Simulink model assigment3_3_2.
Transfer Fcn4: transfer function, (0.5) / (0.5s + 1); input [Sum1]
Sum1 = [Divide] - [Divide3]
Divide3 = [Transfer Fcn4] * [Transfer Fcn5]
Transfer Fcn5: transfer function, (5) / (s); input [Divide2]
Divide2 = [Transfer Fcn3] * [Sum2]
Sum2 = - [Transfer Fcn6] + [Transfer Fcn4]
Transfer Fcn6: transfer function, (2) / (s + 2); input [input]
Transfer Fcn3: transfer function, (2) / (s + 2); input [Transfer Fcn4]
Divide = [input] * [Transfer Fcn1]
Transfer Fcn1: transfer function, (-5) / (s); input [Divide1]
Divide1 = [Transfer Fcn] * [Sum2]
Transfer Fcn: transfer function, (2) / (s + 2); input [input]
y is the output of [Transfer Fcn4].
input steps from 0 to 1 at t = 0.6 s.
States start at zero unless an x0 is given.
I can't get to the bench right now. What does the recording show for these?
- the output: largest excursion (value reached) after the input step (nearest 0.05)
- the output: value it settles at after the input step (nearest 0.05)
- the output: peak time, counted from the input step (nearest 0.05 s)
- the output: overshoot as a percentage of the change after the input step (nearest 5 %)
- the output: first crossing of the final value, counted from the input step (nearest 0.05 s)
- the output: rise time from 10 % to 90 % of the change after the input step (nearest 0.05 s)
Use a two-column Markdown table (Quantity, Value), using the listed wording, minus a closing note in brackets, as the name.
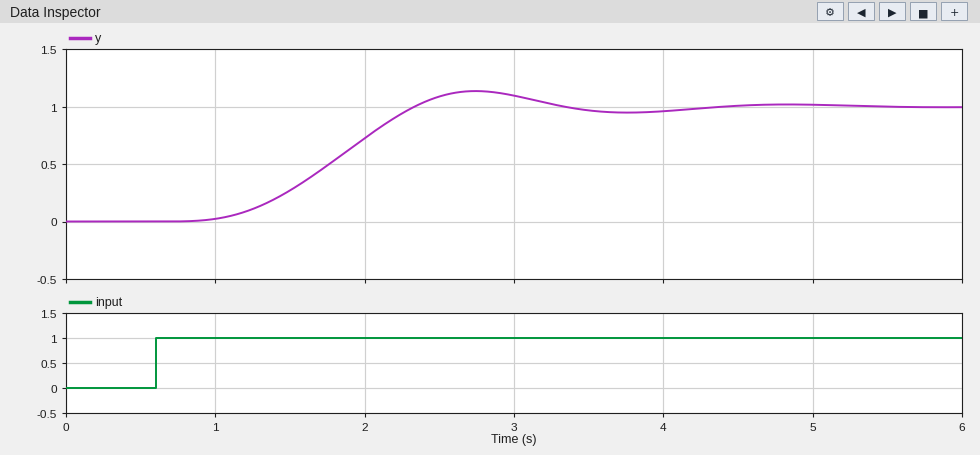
| Quantity | Value |
|---|---|
| the output: largest excursion (value reached) after the input step | 1.15 |
| the output: value it settles at after the input step | 1.00 |
| the output: peak time, counted from the input step | 2.15 s |
| the output: overshoot as a percentage of the change after the input step | 15 % |
| the output: first crossing of the final value, counted from the input step | 1.75 s |
| the output: rise time from 10 % to 90 % of the change after the input step | 0.95 s |
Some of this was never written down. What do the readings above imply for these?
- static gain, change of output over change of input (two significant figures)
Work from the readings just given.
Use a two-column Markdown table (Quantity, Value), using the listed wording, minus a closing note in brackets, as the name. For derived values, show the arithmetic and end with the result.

| Quantity | Value |
|---|---|
| static gain, change of output over change of input | (1 - 0) / (1 - 0) = 1.0 |
